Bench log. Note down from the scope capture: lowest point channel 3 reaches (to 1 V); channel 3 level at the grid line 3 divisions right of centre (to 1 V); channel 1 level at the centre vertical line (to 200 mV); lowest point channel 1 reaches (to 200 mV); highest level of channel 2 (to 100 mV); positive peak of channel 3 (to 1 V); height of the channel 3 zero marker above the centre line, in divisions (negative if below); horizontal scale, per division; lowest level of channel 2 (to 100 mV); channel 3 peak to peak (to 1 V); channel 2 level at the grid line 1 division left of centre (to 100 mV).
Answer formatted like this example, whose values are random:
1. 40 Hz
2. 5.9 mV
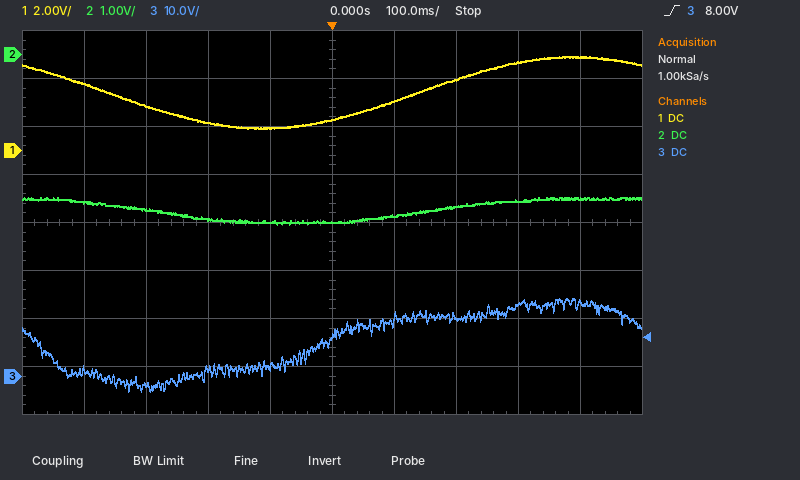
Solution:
1. -3 V
2. 15 V
3. 1.2 V
4. 1.0 V
5. -3.0 V
6. 16 V
7. -3.2 div
8. 100 ms
9. -3.5 V
10. 19 V
11. -3.5 V
